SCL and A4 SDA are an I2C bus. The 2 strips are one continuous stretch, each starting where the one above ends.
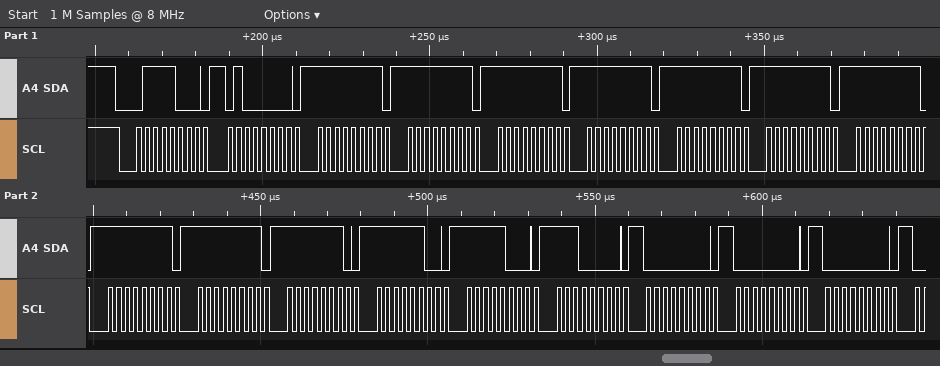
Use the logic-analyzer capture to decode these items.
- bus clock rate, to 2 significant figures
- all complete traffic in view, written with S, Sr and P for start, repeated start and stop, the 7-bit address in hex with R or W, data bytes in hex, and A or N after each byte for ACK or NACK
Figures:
400 kHz
S 3CW A 40 A FF A FF A FF A FF A FF A FF A FF A FF A FF A FE A FC A F8 A E0 A 00 A 00 A 00 A
